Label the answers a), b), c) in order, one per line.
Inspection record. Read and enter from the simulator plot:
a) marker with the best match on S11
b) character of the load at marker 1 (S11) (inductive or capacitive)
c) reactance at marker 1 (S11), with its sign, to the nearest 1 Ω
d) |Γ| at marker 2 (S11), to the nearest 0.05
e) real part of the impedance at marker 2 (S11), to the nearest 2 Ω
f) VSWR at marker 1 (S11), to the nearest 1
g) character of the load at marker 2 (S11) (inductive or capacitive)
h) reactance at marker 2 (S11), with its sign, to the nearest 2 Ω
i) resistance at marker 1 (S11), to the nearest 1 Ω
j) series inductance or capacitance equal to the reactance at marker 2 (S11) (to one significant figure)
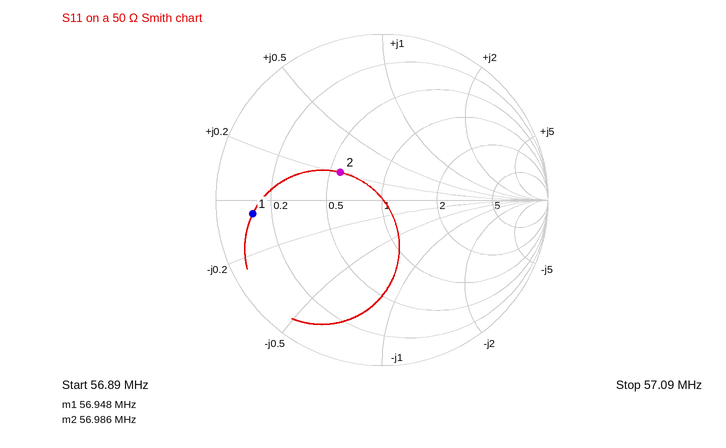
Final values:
a) marker 2
b) capacitive
c) -3 Ω
d) 0.30
e) 28 Ω
f) 8
g) inductive
h) +10 Ω
i) 6 Ω
j) 30 nH
